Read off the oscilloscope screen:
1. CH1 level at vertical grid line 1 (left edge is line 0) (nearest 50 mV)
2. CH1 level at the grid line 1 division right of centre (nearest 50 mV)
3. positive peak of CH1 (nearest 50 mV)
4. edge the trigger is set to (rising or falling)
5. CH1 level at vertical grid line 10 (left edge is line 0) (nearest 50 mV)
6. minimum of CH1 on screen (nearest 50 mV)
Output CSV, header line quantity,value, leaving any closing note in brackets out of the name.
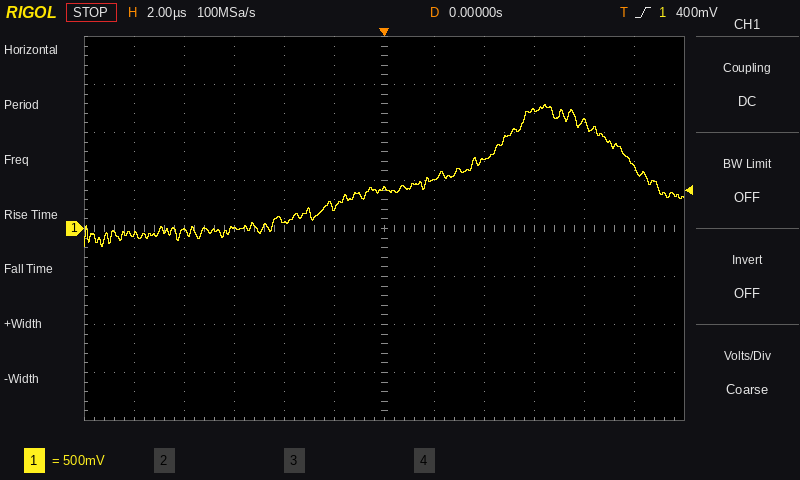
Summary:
quantity,value
CH1 level at vertical grid line 1 (left edge is line 0),-50 mV
CH1 level at the grid line 1 division right of centre,500 mV
positive peak of CH1,1.30 V
edge the trigger is set to,rising
CH1 level at vertical grid line 10 (left edge is line 0),1.10 V
minimum of CH1 on screen,-200 mV
